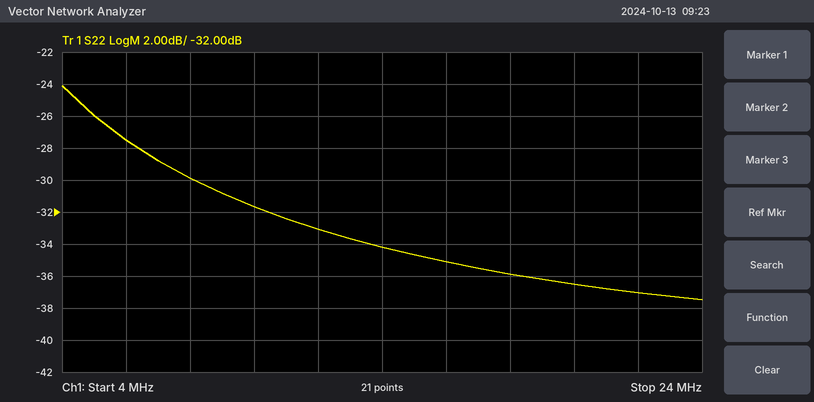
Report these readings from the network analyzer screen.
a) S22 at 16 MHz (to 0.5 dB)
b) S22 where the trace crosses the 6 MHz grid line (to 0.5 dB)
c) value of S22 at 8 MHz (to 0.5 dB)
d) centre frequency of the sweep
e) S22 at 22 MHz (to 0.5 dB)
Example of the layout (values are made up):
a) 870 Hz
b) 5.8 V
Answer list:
a) -35.0 dB
b) -27.5 dB
c) -30.0 dB
d) 14 MHz
e) -37.0 dB
